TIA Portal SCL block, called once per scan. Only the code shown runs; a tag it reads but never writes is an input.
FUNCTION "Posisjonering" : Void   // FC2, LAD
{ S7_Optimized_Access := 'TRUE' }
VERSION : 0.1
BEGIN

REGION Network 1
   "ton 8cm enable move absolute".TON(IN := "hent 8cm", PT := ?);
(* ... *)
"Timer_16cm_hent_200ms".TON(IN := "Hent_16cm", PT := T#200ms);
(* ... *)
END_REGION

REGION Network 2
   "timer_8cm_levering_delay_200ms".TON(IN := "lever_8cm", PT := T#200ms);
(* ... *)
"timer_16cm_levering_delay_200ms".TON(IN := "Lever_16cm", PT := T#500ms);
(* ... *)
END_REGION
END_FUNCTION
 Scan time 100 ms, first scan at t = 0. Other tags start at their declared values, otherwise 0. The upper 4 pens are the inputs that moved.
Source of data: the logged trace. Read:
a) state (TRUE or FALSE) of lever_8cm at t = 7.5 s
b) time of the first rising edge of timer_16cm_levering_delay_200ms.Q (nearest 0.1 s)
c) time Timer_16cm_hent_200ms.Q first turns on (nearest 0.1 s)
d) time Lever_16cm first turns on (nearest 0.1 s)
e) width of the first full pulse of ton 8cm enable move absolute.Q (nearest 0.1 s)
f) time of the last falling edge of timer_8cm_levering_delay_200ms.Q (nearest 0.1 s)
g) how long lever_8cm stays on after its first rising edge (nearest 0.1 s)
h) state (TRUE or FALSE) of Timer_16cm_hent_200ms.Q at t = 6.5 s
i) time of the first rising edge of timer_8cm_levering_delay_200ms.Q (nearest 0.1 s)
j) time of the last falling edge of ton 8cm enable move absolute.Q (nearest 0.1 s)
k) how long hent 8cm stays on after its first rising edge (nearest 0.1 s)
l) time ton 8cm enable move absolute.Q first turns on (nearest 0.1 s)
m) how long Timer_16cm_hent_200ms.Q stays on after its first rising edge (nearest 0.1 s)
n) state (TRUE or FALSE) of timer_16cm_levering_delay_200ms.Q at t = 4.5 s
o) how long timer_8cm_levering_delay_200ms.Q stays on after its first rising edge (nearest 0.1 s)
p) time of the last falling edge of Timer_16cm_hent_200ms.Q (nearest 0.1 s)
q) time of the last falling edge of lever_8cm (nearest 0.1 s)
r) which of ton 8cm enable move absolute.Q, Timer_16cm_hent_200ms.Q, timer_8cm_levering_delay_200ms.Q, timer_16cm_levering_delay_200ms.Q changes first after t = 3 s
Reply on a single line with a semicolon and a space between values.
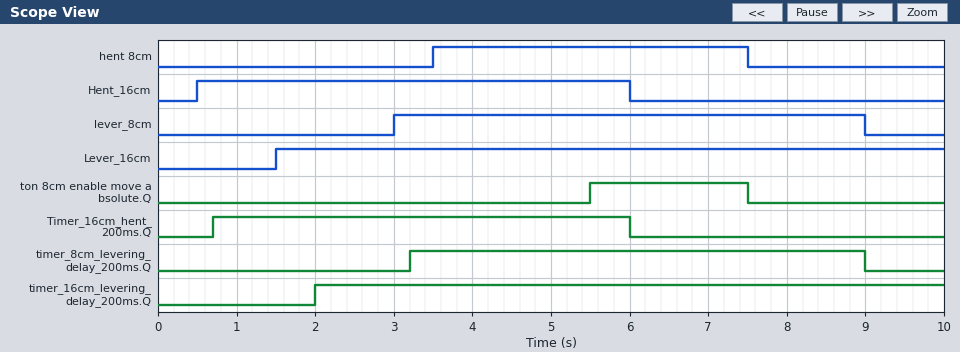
TRUE; 2.0 s; 0.7 s; 1.5 s; 2.0 s; 9.0 s; 6.0 s; FALSE; 3.2 s; 7.5 s; 4.0 s; 5.5 s; 5.3 s; TRUE; 5.8 s; 6.0 s; 9.0 s; timer_8cm_levering_delay_200ms.Q
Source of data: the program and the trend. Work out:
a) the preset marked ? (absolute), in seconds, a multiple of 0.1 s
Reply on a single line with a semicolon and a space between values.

2.0 s
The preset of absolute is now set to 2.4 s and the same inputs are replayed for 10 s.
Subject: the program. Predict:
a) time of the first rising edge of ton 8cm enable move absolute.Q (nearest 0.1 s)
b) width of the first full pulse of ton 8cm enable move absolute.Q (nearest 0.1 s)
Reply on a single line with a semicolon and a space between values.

5.9 s; 1.6 s
